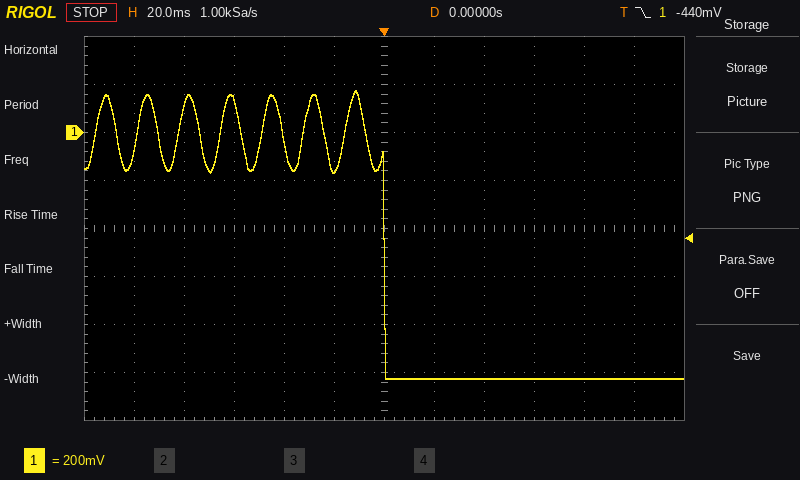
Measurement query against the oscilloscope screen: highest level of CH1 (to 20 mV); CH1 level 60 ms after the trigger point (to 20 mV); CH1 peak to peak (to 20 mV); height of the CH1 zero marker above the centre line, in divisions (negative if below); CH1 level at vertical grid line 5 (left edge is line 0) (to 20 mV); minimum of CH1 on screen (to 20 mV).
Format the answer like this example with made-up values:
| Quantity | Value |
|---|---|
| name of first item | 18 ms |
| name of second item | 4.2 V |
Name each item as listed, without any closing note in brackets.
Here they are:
| Quantity | Value |
|---|---|
| highest level of CH1 | 180 mV |
| CH1 level 60 ms after the trigger point | -1.02 V |
| CH1 peak to peak | 1.20 V |
| height of the CH1 zero marker above the centre line, in divisions | +2.0 div |
| CH1 level at vertical grid line 5 (left edge is line 0) | -160 mV |
| minimum of CH1 on screen | -1.02 V |
